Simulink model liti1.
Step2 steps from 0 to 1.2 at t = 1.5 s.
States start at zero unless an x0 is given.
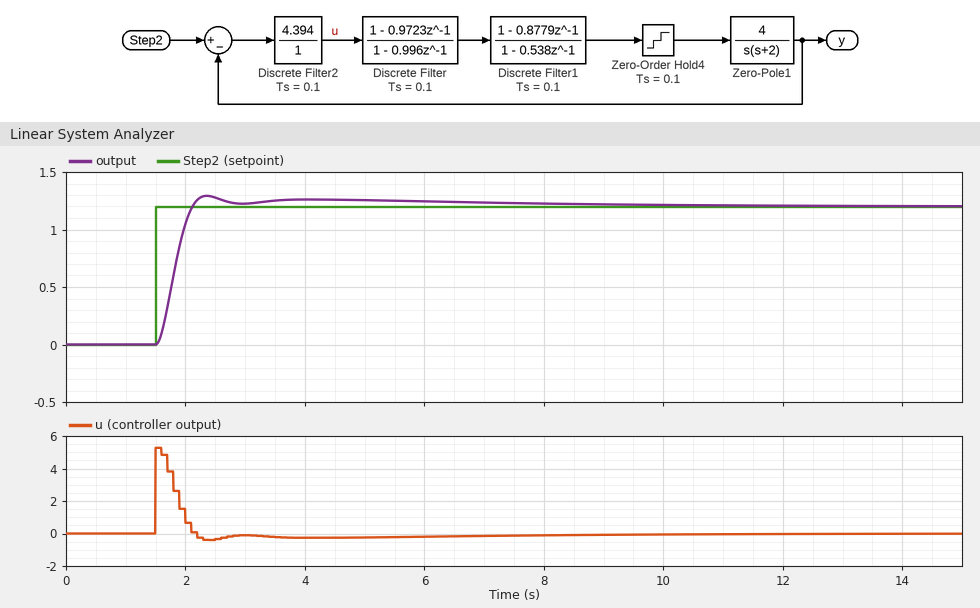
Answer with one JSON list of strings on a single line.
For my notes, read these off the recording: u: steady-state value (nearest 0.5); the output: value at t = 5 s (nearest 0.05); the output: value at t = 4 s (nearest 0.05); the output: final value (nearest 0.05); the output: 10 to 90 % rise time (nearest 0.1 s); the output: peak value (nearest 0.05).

["0.0", "1.25", "1.25", "1.20", "0.4 s", "1.30"]
